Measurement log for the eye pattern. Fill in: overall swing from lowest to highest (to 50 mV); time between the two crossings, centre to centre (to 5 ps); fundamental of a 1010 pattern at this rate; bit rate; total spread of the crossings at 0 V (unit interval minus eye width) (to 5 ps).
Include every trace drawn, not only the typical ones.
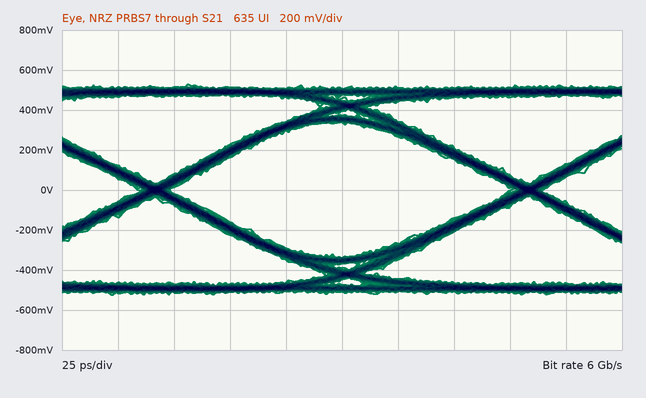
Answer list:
1.05 V
165 ps
3 GHz
6 Gb/s
15 ps
